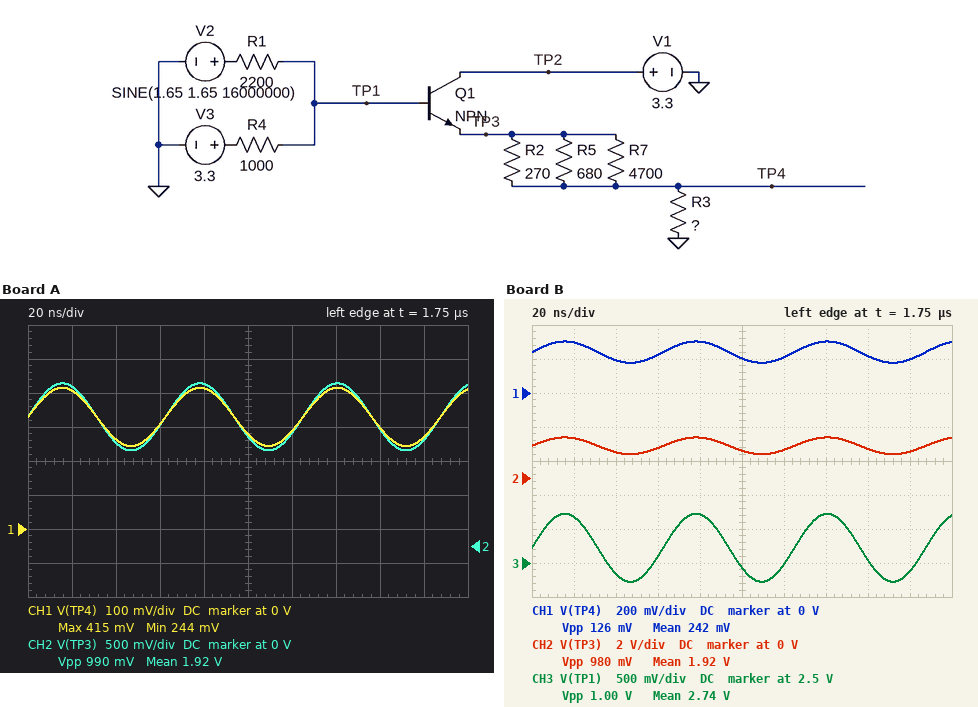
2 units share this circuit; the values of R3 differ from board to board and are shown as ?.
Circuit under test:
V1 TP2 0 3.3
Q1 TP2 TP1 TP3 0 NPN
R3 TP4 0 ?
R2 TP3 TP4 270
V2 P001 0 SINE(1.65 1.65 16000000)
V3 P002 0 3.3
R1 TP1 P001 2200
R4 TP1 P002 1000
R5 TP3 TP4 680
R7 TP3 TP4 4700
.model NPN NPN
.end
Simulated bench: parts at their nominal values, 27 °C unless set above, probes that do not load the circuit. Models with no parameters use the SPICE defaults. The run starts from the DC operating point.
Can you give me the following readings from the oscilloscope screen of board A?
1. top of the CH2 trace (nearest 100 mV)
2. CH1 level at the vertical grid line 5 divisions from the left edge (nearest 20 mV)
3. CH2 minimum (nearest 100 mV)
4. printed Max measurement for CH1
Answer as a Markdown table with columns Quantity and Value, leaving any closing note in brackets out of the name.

| Quantity | Value |
|---|---|
| top of the CH2 trace | 2.4 V |
| CH1 level at the vertical grid line 5 divisions from the left edge | 280 mV |
| CH2 minimum | 1.4 V |
| printed Max measurement for CH1 | 415 mV |
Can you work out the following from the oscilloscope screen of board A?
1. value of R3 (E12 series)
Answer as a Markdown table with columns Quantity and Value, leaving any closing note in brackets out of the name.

| Quantity | Value |
|---|---|
| value of R3 | 39 Ω |
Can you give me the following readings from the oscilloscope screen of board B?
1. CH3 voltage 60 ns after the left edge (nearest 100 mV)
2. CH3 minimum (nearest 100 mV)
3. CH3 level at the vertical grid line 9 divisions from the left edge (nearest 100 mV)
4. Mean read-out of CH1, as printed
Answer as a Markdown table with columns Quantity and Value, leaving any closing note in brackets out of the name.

| Quantity | Value |
|---|---|
| CH3 voltage 60 ns after the left edge | 2.6 V |
| CH3 minimum | 2.2 V |
| CH3 level at the vertical grid line 9 divisions from the left edge | 2.4 V |
| Mean read-out of CH1, as printed | 242 mV |
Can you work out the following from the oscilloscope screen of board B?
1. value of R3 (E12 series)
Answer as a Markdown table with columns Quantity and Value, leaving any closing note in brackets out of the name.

| Quantity | Value |
|---|---|
| value of R3 | 27 Ω |
